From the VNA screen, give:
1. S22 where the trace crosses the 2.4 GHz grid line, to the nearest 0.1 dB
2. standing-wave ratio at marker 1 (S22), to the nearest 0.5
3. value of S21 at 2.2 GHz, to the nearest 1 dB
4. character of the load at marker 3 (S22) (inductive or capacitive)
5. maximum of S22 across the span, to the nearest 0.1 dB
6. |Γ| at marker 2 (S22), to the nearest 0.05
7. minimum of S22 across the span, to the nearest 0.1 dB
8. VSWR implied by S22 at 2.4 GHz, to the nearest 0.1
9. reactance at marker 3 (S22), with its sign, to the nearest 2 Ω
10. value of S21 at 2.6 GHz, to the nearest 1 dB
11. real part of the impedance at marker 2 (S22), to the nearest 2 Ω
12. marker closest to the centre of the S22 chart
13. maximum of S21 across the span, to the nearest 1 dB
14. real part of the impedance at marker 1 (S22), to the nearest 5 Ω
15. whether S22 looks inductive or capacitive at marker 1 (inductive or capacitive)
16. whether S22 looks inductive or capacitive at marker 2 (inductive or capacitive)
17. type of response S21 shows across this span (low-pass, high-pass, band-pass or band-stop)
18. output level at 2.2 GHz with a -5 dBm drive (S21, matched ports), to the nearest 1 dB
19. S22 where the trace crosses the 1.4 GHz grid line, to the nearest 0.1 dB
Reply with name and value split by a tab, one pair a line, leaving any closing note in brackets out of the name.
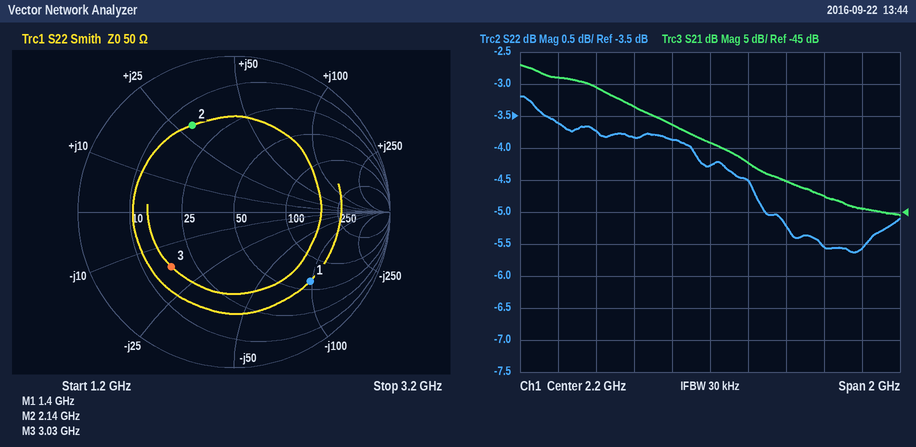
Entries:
S22 where the trace crosses the 2.4 GHz grid line, to the nearest 0.1 dB	-4.5 dB
standing-wave ratio at marker 1 (S22), to the nearest 0.5	5.0
value of S21 at 2.2 GHz, to the nearest 1 dB	-34 dB
character of the load at marker 3 (S22)	capacitive
maximum of S22 across the span, to the nearest 0.1 dB	-3.2 dB
|Γ| at marker 2 (S22), to the nearest 0.05	0.60
minimum of S22 across the span, to the nearest 0.1 dB	-5.6 dB
VSWR implied by S22 at 2.4 GHz, to the nearest 0.1	3.9
reactance at marker 3 (S22), with its sign, to the nearest 2 Ω	-16 Ω
value of S21 at 2.6 GHz, to the nearest 1 dB	-40 dB
real part of the impedance at marker 2 (S22), to the nearest 2 Ω	16 Ω
marker closest to the centre of the S22 chart	marker 3
maximum of S21 across the span, to the nearest 1 dB	-22 dB
real part of the impedance at marker 1 (S22), to the nearest 5 Ω	60 Ω
whether S22 looks inductive or capacitive at marker 1	capacitive
whether S22 looks inductive or capacitive at marker 2	inductive
type of response S21 shows across this span	low-pass
output level at 2.2 GHz with a -5 dBm drive (S21, matched ports), to the nearest 1 dB	-39 dBm
S22 where the trace crosses the 1.4 GHz grid line, to the nearest 0.1 dB	-3.6 dB
